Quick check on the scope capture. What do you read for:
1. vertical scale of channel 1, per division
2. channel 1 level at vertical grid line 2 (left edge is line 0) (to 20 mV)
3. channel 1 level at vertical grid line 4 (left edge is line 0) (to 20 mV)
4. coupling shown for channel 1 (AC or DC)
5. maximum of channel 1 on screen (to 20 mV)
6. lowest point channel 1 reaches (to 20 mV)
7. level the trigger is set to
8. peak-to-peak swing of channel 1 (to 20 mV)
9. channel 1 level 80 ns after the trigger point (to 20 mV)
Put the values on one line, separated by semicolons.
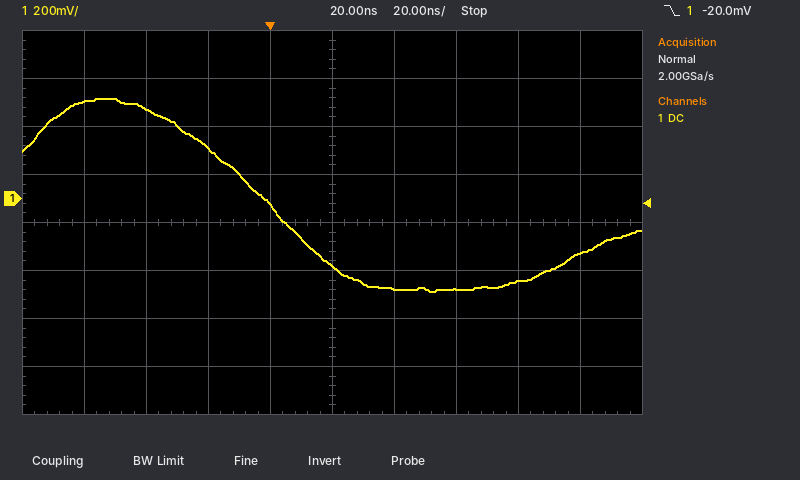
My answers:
200 mV; 380 mV; -20 mV; DC; 420 mV; -380 mV; -20.0 mV; 800 mV; -340 mV
